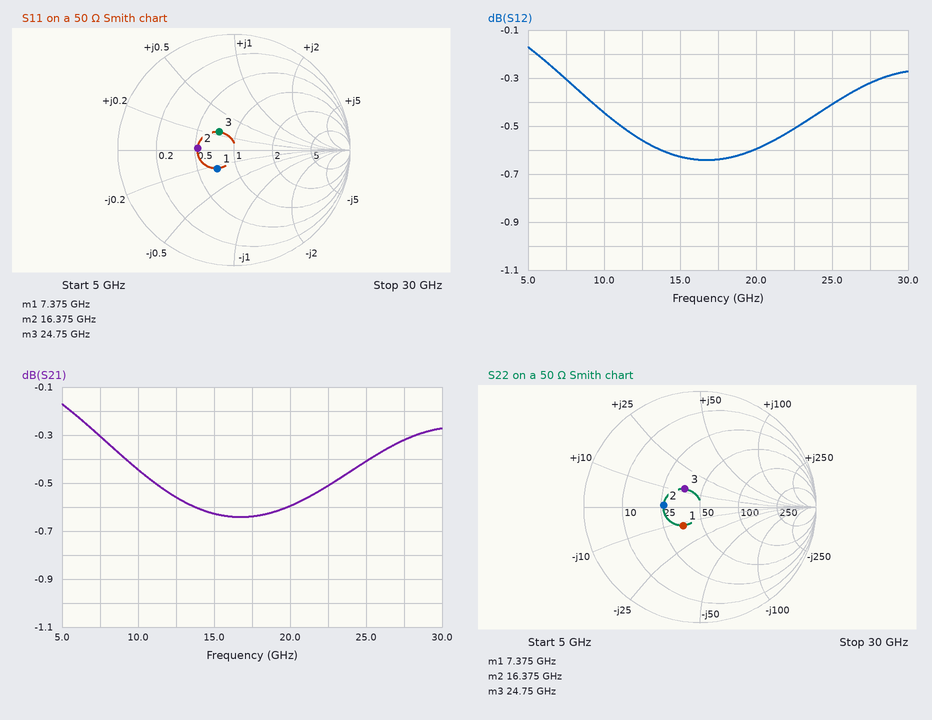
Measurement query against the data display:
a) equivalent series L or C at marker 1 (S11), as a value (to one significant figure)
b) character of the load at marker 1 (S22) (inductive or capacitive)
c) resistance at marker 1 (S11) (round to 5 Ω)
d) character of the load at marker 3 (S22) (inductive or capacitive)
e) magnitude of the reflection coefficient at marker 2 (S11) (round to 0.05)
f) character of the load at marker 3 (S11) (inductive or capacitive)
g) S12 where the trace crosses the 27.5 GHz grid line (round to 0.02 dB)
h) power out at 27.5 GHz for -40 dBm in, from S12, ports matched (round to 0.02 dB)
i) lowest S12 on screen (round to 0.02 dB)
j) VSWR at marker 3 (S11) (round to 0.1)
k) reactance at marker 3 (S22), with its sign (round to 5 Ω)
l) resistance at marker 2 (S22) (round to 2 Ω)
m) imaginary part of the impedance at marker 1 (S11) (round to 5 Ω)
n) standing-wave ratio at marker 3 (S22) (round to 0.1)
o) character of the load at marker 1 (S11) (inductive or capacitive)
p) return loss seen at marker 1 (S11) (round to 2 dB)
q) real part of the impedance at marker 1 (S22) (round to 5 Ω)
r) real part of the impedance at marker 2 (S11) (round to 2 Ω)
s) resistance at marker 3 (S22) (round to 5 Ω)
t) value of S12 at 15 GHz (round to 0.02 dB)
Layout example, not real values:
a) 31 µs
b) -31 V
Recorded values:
a) 2 pF
b) capacitive
c) 35 Ω
d) inductive
e) 0.30
f) inductive
g) -0.32 dB
h) -40.32 dBm
i) -0.64 dB
j) 1.5
k) +10 Ω
l) 26 Ω
m) -10 Ω
n) 1.5
o) capacitive
p) 14 dB
q) 35 Ω
r) 26 Ω
s) 35 Ω
t) -0.62 dB
